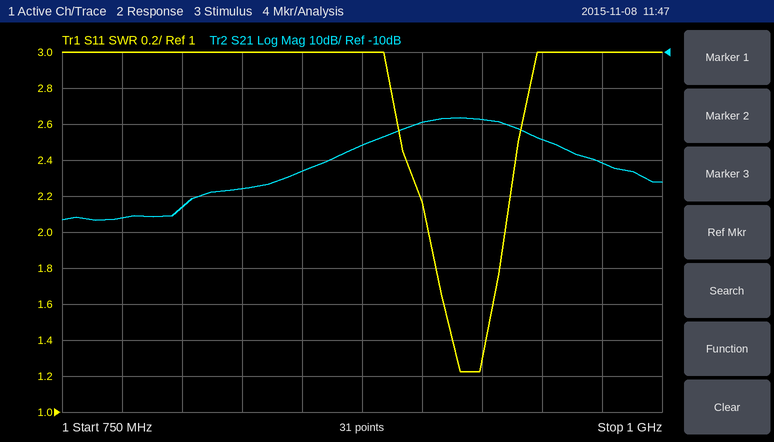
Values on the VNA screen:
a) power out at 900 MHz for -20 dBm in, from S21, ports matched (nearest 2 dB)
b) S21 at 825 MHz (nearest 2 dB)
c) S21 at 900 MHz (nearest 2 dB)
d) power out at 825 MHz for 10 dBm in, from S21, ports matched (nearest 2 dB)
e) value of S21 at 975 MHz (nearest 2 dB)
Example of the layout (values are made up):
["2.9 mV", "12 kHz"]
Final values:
["-50 dBm", "-48 dB", "-30 dB", "-38 dBm", "-40 dB"]
